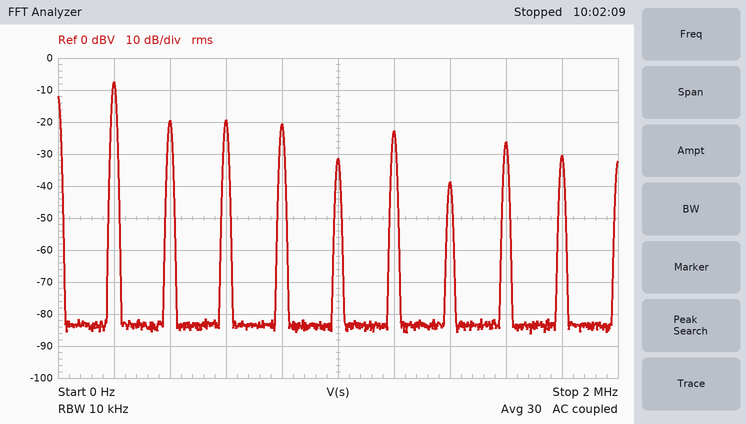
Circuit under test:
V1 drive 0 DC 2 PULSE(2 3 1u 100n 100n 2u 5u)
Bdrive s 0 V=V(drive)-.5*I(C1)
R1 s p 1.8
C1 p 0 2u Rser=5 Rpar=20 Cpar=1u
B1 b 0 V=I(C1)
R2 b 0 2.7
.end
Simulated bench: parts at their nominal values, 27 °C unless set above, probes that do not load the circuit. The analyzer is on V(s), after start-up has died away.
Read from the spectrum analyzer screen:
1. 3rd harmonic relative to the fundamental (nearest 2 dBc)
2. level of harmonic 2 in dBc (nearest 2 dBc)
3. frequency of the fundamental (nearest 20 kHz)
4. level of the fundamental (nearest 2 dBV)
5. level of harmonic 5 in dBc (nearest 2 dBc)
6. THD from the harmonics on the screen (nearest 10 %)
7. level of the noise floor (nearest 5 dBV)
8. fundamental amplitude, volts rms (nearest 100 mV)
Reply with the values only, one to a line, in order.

-12 dBc
-12 dBc
200 kHz
-8 dBV
-24 dBc
50 %
-85 dBV
400 mV
